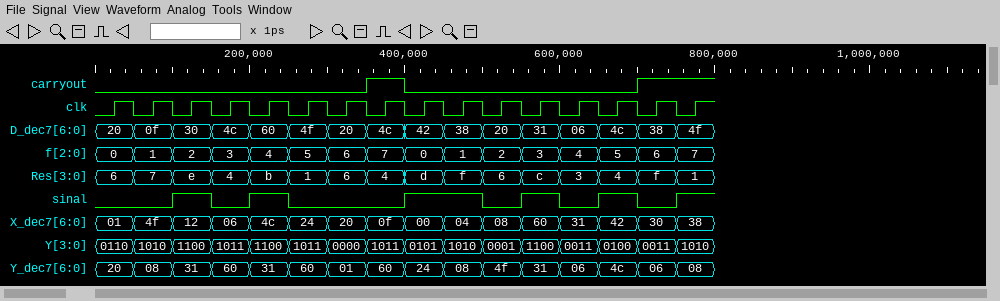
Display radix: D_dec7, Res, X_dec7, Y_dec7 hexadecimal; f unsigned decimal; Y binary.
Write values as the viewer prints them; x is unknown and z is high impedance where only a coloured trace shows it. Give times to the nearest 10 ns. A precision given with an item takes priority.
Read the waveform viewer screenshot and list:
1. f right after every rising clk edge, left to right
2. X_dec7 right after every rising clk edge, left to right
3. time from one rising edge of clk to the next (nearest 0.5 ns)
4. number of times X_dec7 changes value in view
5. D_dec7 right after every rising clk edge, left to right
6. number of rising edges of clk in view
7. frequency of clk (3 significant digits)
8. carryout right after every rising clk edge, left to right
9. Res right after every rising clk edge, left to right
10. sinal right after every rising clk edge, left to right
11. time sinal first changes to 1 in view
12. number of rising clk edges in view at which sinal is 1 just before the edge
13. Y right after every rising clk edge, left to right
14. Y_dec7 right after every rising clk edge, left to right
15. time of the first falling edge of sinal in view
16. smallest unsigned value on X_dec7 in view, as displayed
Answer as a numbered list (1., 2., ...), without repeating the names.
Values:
1. 0, 1, 2, 3, 4, 5, 6, 7, 0, 1, 2, 3, 4, 5, 6, 7
2. 01, 4f, 12, 06, 4c, 24, 20, 0f, 00, 04, 08, 60, 31, 42, 30, 38
3. 50 ns
4. 15
5. 20, 0f, 30, 4c, 60, 4f, 20, 4c, 42, 38, 20, 31, 06, 4c, 38, 4f
6. 16
7. 20.0 MHz
8. 0 0 0 0 0 0 0 1 0 0 0 0 0 0 1 1
9. 6, 7, e, 4, b, 1, 6, 4, d, f, 6, c, 3, 4, f, 1
10. 0 0 1 0 1 0 0 0 1 1 0 1 0 1 0 1
11. 100 ns
12. 7
13. 0110, 1010, 1100, 1011, 1100, 1011, 0000, 1011, 0101, 1010, 0001, 1100, 0011, 0100, 0011, 1010
14. 20, 08, 31, 60, 31, 60, 01, 60, 24, 08, 4f, 31, 06, 4c, 06, 08
15. 150 ns
16. 00
